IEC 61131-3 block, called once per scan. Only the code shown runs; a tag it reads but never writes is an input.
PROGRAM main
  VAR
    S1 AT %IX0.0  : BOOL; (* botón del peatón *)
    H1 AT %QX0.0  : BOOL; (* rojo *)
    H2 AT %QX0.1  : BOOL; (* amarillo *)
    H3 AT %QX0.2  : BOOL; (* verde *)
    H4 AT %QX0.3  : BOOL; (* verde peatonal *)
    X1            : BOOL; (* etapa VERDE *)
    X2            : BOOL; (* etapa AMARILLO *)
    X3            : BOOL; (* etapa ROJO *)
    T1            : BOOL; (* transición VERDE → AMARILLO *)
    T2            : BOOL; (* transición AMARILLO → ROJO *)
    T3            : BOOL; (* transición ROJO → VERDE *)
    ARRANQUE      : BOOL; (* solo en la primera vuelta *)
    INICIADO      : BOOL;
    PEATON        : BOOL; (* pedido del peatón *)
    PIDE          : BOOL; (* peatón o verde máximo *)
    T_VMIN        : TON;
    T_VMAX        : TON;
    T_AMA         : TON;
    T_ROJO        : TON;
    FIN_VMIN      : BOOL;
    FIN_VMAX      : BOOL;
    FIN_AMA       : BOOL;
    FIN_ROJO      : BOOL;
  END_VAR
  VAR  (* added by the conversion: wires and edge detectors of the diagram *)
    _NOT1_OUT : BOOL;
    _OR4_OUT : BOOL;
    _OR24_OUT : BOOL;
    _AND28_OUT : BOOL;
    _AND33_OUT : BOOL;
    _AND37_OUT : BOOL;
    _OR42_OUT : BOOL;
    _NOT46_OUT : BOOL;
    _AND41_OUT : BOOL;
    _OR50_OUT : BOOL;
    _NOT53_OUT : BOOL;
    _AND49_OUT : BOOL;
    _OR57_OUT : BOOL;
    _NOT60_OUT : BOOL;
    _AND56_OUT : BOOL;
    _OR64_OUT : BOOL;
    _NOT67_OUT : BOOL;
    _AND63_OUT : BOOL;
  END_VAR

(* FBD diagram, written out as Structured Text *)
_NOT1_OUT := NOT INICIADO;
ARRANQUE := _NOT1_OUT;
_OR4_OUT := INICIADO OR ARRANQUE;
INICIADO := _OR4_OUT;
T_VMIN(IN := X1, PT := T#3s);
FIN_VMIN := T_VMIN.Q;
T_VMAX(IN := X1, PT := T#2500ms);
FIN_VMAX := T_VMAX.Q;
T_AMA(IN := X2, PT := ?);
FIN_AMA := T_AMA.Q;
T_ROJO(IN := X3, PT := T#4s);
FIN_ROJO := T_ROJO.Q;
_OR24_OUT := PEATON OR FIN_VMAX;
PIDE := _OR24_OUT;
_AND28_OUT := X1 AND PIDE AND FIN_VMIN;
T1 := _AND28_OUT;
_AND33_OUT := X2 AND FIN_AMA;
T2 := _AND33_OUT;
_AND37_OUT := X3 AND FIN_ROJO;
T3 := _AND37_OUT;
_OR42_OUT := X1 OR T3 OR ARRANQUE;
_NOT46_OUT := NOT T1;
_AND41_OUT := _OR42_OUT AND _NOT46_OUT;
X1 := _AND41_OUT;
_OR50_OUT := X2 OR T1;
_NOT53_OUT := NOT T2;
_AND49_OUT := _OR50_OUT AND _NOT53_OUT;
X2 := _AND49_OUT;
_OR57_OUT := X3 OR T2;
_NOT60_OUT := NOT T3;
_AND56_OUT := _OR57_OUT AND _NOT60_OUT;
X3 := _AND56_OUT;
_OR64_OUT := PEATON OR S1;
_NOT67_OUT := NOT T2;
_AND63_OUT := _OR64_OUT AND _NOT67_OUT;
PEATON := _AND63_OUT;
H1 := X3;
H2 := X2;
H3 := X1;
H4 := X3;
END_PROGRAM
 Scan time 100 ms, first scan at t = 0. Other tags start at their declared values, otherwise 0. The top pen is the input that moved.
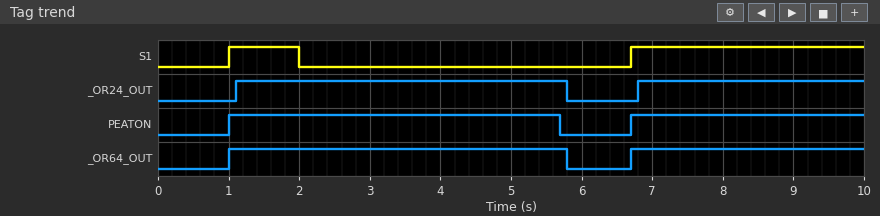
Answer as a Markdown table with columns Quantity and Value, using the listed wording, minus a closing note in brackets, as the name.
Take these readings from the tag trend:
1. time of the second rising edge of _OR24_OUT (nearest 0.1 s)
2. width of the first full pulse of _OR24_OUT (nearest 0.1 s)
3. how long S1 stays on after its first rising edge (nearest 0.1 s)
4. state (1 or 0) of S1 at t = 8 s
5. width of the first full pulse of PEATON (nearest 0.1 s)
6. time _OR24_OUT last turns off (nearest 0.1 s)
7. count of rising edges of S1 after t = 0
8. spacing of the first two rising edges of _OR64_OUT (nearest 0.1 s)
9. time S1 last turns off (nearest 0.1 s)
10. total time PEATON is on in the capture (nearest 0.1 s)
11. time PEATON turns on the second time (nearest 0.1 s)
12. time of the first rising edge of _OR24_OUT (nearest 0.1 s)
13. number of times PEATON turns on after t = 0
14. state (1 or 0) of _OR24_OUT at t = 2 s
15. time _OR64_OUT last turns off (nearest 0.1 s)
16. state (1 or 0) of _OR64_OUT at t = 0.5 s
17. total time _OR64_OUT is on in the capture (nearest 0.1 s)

| Quantity | Value |
|---|---|
| time of the second rising edge of _OR24_OUT | 6.8 s |
| width of the first full pulse of _OR24_OUT | 4.7 s |
| how long S1 stays on after its first rising edge | 1.0 s |
| state (1 or 0) of S1 at t = 8 s | 1 |
| width of the first full pulse of PEATON | 4.7 s |
| time _OR24_OUT last turns off | 5.8 s |
| count of rising edges of S1 after t = 0 | 2 |
| spacing of the first two rising edges of _OR64_OUT | 5.7 s |
| time S1 last turns off | 2.0 s |
| total time PEATON is on in the capture | 8.0 s |
| time PEATON turns on the second time | 6.7 s |
| time of the first rising edge of _OR24_OUT | 1.1 s |
| number of times PEATON turns on after t = 0 | 2 |
| state (1 or 0) of _OR24_OUT at t = 2 s | 1 |
| time _OR64_OUT last turns off | 5.8 s |
| state (1 or 0) of _OR64_OUT at t = 0.5 s | 0 |
| total time _OR64_OUT is on in the capture | 8.1 s |
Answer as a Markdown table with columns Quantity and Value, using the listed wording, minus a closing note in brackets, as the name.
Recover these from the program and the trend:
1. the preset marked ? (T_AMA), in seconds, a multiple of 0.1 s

| Quantity | Value |
|---|---|
| the preset marked ? (T_AMA), in seconds, a multiple of 0.1 s | 2.5 s |
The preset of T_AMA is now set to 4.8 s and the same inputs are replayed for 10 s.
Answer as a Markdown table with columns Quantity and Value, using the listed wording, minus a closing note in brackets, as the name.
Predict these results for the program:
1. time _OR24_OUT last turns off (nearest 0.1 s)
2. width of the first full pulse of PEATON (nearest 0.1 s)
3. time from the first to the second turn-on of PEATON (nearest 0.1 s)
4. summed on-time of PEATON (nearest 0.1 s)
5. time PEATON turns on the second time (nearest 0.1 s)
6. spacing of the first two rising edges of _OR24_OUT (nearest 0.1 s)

| Quantity | Value |
|---|---|
| time _OR24_OUT last turns off | 8.1 s |
| width of the first full pulse of PEATON | 7.0 s |
| time from the first to the second turn-on of PEATON | 7.1 s |
| summed on-time of PEATON | 8.9 s |
| time PEATON turns on the second time | 8.1 s |
| spacing of the first two rising edges of _OR24_OUT | 7.1 s |
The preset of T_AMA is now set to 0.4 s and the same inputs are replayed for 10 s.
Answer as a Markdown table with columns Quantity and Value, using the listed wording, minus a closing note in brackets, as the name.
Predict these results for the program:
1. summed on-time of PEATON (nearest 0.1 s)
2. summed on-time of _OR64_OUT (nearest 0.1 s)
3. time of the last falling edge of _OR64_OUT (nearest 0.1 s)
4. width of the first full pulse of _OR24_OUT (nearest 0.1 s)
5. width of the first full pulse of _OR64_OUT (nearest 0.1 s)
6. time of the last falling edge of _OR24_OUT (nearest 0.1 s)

| Quantity | Value |
|---|---|
| summed on-time of PEATON | 5.9 s |
| summed on-time of _OR64_OUT | 6.0 s |
| time of the last falling edge of _OR64_OUT | 3.7 s |
| width of the first full pulse of _OR24_OUT | 2.6 s |
| width of the first full pulse of _OR64_OUT | 2.7 s |
| time of the last falling edge of _OR24_OUT | 3.7 s |
